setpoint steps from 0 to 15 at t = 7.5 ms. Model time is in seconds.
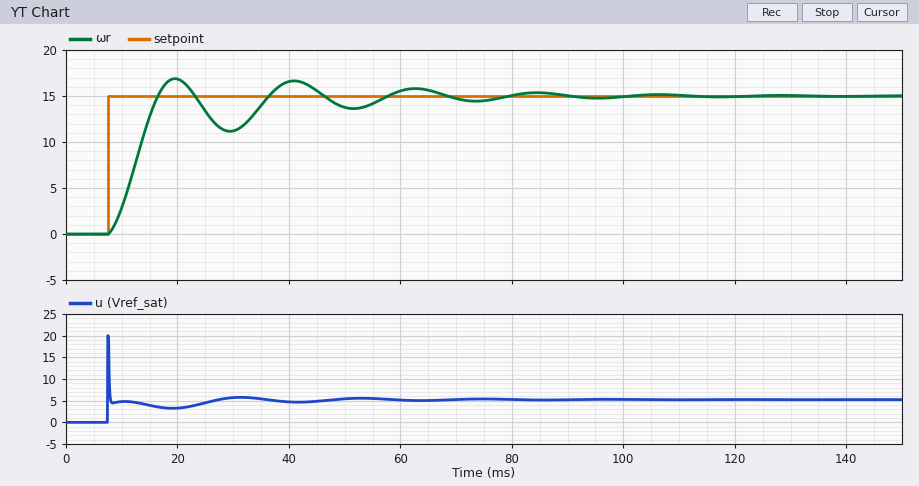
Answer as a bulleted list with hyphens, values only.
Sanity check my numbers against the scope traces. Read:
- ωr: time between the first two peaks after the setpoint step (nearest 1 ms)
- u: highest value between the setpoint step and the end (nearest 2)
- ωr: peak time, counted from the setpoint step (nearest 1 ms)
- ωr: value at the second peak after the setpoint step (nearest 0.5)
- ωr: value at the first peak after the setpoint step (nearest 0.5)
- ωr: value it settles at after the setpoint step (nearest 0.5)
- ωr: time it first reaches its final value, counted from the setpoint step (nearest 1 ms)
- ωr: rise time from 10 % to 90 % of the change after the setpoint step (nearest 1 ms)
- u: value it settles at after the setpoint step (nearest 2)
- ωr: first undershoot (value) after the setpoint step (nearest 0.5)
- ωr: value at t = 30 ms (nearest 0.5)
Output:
- 21 ms
- 20
- 12 ms
- 16.5
- 17.0
- 15.0
- 9 ms
- 6 ms
- 6
- 11.0
- 11.0
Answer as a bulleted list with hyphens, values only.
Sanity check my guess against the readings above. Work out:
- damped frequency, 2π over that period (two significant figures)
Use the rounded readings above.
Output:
- 0.30 rad/ms
